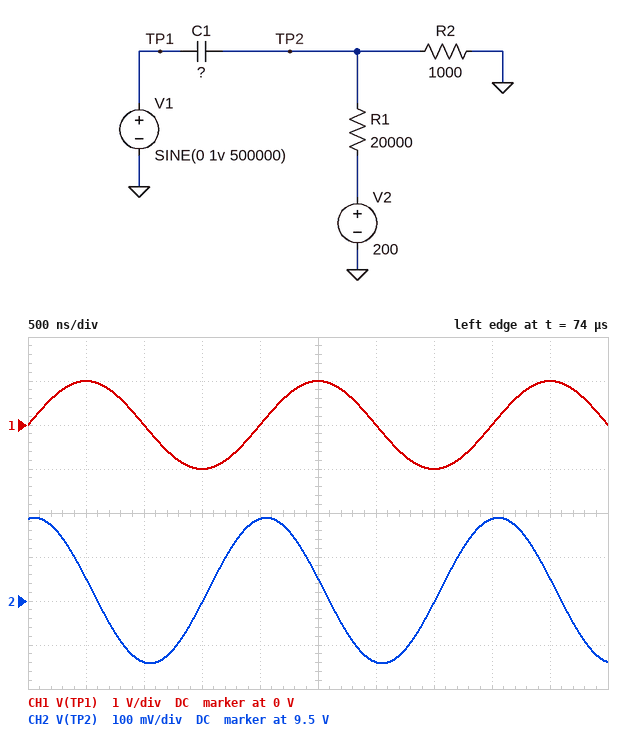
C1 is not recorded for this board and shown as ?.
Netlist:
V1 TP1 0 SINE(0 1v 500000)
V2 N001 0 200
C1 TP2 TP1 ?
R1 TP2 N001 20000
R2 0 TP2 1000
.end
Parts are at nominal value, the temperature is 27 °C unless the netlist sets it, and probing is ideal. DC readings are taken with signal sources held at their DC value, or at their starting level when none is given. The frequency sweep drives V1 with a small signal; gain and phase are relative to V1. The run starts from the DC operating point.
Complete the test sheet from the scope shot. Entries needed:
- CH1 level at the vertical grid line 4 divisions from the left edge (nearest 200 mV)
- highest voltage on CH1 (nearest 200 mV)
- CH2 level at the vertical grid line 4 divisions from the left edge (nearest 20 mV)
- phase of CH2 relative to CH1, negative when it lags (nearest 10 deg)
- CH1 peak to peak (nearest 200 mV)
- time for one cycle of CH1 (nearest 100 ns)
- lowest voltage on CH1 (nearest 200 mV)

0 V
1.0 V
9.68 V
80 deg
2.0 V
2.0 µs
-1.0 V
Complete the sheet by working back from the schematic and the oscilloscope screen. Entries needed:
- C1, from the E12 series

56 pF
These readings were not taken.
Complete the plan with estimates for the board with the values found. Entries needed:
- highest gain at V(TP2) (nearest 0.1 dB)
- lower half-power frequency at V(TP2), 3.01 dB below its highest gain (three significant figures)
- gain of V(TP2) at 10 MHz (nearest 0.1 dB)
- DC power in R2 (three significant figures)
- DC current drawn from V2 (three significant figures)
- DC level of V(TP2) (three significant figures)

0 dB
2.98 MHz
-0.4 dB
90.7 mW
9.52 mA
9.52 V
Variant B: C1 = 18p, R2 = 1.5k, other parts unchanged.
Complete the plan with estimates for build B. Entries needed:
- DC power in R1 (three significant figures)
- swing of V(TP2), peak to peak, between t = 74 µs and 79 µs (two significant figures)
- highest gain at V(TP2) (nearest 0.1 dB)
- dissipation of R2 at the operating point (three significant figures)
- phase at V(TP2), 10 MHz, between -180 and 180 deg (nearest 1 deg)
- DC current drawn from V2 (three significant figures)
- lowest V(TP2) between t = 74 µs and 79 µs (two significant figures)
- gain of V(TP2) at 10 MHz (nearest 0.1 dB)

1.73 W
160 mV
0 dB
130 mW
32 deg
9.30 mA
14 V
-1.5 dB
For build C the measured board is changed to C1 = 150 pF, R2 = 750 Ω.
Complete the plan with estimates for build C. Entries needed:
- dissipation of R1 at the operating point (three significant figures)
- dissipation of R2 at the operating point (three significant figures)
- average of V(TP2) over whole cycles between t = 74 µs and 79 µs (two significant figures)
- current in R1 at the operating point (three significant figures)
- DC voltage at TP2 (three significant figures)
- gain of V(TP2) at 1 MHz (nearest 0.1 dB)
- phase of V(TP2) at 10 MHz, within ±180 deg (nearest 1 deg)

1.86 W
69.7 mW
7.2 V
9.64 mA
7.23 V
-5.0 dB
8 deg
